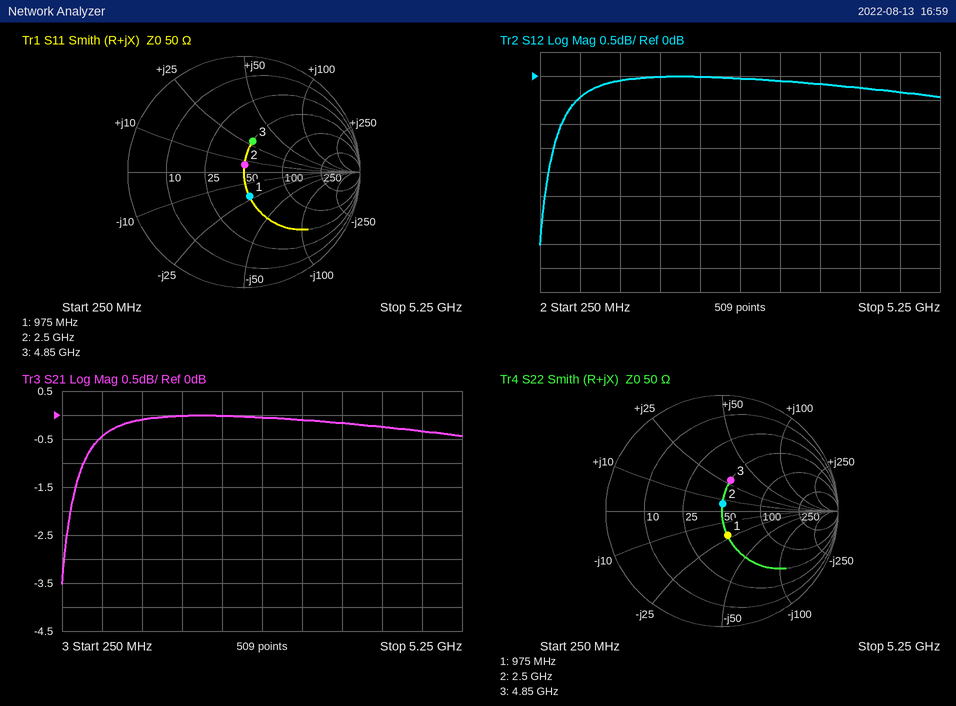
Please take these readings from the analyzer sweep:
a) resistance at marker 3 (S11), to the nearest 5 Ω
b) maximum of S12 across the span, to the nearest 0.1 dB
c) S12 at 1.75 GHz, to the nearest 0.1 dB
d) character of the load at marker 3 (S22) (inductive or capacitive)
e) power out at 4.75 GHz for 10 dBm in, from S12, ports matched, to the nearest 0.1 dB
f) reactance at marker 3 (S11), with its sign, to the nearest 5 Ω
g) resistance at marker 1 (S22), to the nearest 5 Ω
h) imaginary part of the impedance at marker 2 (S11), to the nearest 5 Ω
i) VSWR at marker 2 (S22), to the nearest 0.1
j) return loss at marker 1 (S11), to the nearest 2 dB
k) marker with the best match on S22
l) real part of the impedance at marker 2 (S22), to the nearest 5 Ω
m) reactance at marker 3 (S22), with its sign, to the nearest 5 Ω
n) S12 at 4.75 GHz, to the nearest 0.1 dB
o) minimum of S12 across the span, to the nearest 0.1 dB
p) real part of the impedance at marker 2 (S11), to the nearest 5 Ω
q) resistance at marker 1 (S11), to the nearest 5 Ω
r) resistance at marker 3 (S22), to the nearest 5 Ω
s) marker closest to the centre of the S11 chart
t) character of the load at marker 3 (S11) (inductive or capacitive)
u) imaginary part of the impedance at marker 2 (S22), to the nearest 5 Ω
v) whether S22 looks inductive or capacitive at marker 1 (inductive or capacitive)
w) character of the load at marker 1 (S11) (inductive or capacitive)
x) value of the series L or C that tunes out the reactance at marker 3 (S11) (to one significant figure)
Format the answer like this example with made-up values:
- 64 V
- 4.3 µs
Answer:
- 50 Ω
- 0.0 dB
- 0.0 dB
- inductive
- 9.7 dBm
- +30 Ω
- 50 Ω
- +5 Ω
- 1.1
- 14 dB
- marker 2
- 50 Ω
- +30 Ω
- -0.3 dB
- -3.5 dB
- 50 Ω
- 50 Ω
- 50 Ω
- marker 2
- inductive
- +5 Ω
- capacitive
- capacitive
- 1 pF
